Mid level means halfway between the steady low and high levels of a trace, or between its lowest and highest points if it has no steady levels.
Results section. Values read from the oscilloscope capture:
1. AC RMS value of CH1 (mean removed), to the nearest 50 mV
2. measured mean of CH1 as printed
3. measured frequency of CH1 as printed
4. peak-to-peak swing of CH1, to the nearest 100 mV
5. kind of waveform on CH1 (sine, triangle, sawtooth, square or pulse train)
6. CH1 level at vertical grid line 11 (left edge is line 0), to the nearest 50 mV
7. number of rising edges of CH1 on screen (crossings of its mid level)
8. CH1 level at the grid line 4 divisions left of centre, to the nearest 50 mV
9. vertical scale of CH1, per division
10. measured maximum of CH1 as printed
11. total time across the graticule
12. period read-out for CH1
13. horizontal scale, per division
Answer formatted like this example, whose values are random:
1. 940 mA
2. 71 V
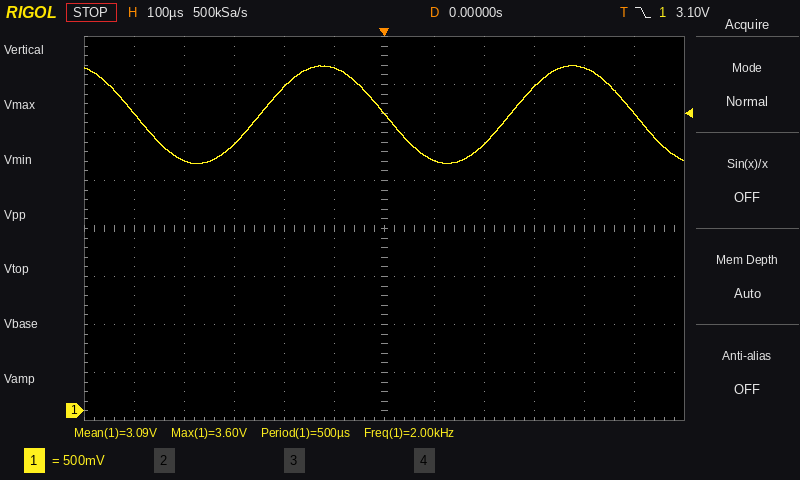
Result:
1. 350 mV
2. 3.09 V
3. 2.00 kHz
4. 1.00 V
5. sine
6. 3.10 V
7. 2
8. 2.60 V
9. 500 mV
10. 3.60 V
11. 1.2 ms
12. 500 µs
13. 100 µs
